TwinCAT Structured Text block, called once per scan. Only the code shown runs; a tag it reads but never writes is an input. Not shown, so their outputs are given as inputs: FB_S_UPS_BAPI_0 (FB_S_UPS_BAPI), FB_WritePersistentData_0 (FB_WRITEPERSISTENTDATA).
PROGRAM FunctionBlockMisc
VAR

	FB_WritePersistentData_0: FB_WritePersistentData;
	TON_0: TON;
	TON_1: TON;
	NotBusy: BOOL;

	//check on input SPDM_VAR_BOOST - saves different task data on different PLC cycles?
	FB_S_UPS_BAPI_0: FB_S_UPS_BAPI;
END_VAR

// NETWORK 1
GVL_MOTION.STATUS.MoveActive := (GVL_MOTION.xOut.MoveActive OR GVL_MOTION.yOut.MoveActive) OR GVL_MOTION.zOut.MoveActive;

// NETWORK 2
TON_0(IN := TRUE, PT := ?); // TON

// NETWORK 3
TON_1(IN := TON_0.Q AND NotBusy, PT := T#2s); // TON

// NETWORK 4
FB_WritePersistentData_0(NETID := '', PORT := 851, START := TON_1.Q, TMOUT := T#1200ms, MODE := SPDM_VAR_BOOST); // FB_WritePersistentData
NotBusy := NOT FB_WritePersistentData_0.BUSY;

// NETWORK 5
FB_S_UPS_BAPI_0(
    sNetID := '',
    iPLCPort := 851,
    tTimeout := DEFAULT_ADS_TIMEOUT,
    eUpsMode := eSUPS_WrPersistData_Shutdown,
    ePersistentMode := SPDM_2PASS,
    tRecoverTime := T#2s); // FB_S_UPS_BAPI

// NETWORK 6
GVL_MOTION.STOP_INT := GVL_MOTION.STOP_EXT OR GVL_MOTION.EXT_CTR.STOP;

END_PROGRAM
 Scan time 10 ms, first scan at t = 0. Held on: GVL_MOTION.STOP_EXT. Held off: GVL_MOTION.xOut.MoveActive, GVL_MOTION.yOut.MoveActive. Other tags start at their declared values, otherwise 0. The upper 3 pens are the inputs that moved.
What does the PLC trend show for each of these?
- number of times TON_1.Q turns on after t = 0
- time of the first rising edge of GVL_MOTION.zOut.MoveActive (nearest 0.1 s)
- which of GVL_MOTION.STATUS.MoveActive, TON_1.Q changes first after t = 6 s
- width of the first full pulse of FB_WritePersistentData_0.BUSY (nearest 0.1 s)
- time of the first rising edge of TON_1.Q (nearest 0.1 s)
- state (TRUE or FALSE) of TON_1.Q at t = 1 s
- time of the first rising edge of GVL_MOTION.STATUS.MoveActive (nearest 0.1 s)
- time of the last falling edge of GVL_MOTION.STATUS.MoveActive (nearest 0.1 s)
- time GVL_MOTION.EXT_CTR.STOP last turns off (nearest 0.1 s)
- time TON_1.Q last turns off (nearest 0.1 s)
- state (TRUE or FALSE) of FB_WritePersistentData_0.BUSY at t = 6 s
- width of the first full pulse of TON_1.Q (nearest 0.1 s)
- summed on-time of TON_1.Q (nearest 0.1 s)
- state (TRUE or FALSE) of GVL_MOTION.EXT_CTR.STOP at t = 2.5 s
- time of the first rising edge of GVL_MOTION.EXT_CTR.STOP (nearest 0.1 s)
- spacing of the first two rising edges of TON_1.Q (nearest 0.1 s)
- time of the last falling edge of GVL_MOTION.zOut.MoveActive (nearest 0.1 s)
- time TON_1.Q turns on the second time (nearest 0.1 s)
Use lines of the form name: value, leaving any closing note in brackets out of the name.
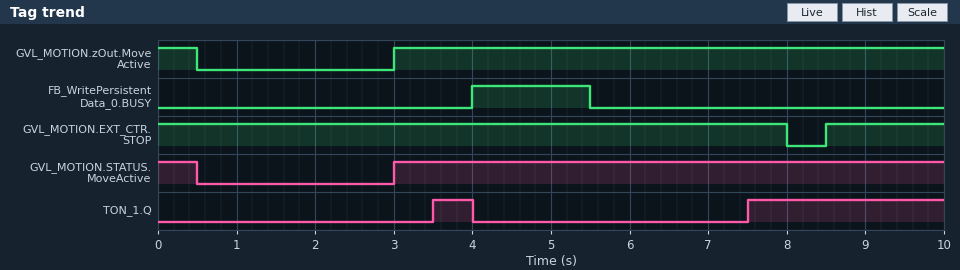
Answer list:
number of times TON_1.Q turns on after t = 0: 2
time of the first rising edge of GVL_MOTION.zOut.MoveActive: 3.0 s
which of GVL_MOTION.STATUS.MoveActive, TON_1.Q changes first after t = 6 s: TON_1.Q
width of the first full pulse of FB_WritePersistentData_0.BUSY: 1.5 s
time of the first rising edge of TON_1.Q: 3.5 s
state (TRUE or FALSE) of TON_1.Q at t = 1 s: FALSE
time of the first rising edge of GVL_MOTION.STATUS.MoveActive: 3.0 s
time of the last falling edge of GVL_MOTION.STATUS.MoveActive: 0.5 s
time GVL_MOTION.EXT_CTR.STOP last turns off: 8.0 s
time TON_1.Q last turns off: 4.0 s
state (TRUE or FALSE) of FB_WritePersistentData_0.BUSY at t = 6 s: FALSE
width of the first full pulse of TON_1.Q: 0.5 s
summed on-time of TON_1.Q: 3.0 s
state (TRUE or FALSE) of GVL_MOTION.EXT_CTR.STOP at t = 2.5 s: TRUE
time of the first rising edge of GVL_MOTION.EXT_CTR.STOP: 8.5 s
spacing of the first two rising edges of TON_1.Q: 4.0 s
time of the last falling edge of GVL_MOTION.zOut.MoveActive: 0.5 s
time TON_1.Q turns on the second time: 7.5 s
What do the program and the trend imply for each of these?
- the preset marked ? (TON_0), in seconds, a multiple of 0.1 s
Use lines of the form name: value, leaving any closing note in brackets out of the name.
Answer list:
the preset marked ? (TON_0), in seconds, a multiple of 0.1 s: 1.5 s
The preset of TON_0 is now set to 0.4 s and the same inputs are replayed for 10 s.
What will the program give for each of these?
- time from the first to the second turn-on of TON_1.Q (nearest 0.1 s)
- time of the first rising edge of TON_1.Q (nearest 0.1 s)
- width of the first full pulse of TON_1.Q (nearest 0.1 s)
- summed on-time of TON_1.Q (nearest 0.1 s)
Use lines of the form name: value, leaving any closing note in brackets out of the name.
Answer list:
time from the first to the second turn-on of TON_1.Q: 5.1 s
time of the first rising edge of TON_1.Q: 2.4 s
width of the first full pulse of TON_1.Q: 1.6 s
summed on-time of TON_1.Q: 4.1 s
